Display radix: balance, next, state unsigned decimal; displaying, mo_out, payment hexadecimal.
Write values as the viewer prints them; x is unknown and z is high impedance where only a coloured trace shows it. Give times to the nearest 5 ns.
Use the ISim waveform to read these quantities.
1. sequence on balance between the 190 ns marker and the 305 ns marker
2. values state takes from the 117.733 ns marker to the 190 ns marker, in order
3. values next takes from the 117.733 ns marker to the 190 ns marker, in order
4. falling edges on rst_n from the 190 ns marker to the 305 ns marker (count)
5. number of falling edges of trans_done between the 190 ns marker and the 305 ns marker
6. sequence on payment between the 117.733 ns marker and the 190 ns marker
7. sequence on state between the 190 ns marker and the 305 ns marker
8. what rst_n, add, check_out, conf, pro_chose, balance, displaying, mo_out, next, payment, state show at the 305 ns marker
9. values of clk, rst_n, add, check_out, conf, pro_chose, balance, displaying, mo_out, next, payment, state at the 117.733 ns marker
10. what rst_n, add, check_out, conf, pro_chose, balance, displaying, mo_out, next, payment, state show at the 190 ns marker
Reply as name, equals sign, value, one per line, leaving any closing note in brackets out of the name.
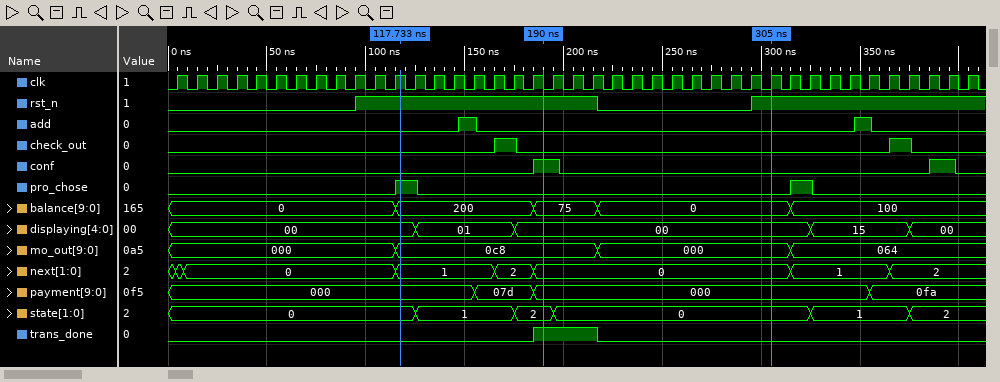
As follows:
sequence on balance between the 190 ns marker and the 305 ns marker = 75, 0
values state takes from the 117.733 ns marker to the 190 ns marker, in order = 0, 1, 2
values next takes from the 117.733 ns marker to the 190 ns marker, in order = 1, 2, 0
falling edges on rst_n from the 190 ns marker to the 305 ns marker = 1
number of falling edges of trans_done between the 190 ns marker and the 305 ns marker = 1
sequence on payment between the 117.733 ns marker and the 190 ns marker = 000, 07d, 000
sequence on state between the 190 ns marker and the 305 ns marker = 2, 0
what rst_n, add, check_out, conf, pro_chose, balance, displaying, mo_out, next, payment, state show at the 305 ns marker = rst_n=1, add=0, check_out=0, conf=0, pro_chose=0, balance=0, displaying=00, mo_out=000, next=0, payment=000, state=0
values of clk, rst_n, add, check_out, conf, pro_chose, balance, displaying, mo_out, next, payment, state at the 117.733 ns marker = clk=1, rst_n=1, add=0, check_out=0, conf=0, pro_chose=1, balance=200, displaying=00, mo_out=0c8, next=1, payment=000, state=0
what rst_n, add, check_out, conf, pro_chose, balance, displaying, mo_out, next, payment, state show at the 190 ns marker = rst_n=1, add=0, check_out=0, conf=1, pro_chose=0, balance=75, displaying=00, mo_out=0c8, next=0, payment=000, state=2
